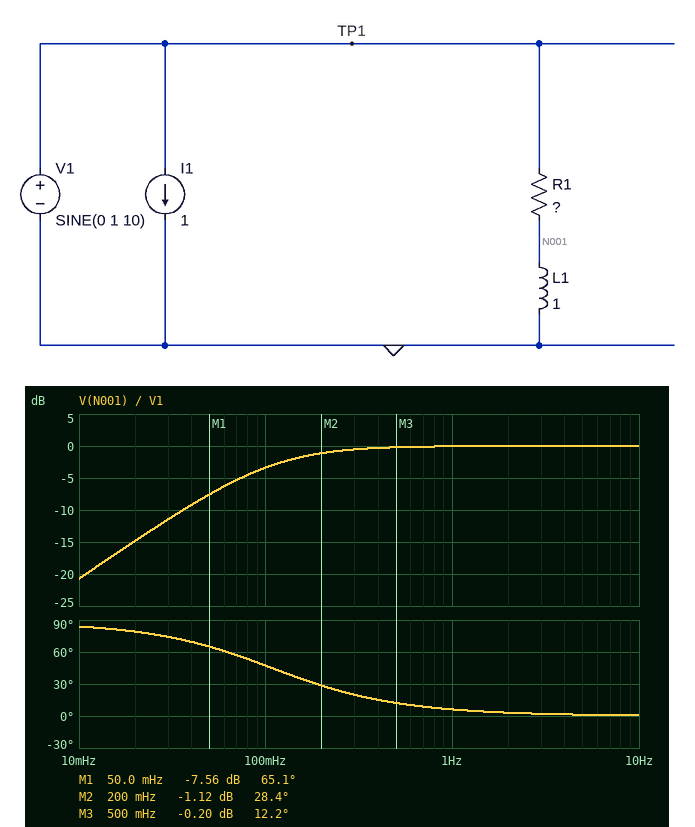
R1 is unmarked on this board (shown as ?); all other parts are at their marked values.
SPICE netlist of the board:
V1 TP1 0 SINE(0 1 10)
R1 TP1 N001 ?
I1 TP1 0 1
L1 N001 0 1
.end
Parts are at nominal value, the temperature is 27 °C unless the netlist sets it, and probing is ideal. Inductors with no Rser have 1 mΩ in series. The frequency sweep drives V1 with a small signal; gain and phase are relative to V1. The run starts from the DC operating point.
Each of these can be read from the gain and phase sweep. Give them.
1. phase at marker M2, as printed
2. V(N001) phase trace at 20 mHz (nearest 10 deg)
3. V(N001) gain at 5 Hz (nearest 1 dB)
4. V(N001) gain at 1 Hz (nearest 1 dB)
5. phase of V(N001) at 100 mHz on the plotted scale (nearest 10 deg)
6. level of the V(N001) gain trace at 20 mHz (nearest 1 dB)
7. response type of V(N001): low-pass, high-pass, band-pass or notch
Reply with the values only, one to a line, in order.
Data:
28.4 deg
80 deg
0 dB
0 dB
50 deg
-15 dB
high-pass
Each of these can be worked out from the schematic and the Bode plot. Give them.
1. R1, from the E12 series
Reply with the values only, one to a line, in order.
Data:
0.68 Ω
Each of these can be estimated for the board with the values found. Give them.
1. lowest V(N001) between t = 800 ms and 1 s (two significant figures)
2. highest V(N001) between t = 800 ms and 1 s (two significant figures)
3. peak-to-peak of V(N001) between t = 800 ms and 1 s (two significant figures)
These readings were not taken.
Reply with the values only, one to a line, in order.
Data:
-1.0 V
990 mV
2.0 V
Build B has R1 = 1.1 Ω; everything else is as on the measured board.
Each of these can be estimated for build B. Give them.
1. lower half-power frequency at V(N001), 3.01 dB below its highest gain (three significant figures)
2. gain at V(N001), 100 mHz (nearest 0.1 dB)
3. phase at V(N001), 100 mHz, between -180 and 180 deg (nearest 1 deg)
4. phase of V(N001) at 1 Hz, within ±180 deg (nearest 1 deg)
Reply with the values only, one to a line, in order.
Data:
175 mHz
-6.1 dB
60 deg
10 deg
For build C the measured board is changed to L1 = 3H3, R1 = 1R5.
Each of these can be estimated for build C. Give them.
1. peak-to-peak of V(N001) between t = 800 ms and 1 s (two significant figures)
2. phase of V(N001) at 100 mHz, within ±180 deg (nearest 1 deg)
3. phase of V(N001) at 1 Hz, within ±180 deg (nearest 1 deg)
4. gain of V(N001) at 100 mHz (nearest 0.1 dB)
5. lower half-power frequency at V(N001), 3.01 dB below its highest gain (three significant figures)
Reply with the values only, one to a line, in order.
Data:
2.0 V
36 deg
4 deg
-1.8 dB
72.4 mHz
